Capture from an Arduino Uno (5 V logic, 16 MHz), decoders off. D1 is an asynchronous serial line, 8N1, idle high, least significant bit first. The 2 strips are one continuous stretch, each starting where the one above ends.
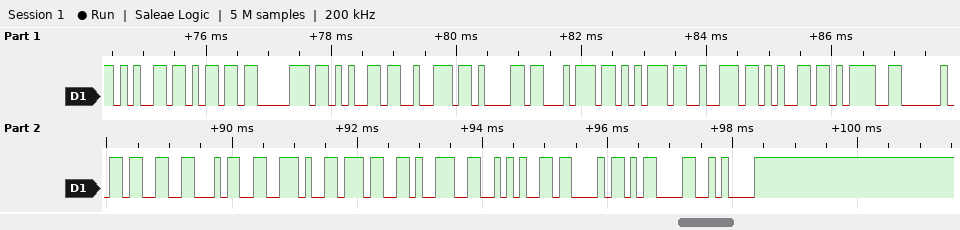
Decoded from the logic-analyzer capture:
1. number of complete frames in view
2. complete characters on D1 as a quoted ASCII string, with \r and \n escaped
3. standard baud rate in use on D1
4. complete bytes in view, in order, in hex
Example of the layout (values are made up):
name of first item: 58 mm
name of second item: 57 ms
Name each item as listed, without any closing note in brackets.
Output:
number of complete frames in view: 21
complete characters on D1 as a quoted ASCII string, with \r and \n escaped: "emperature= 34.79*C\r\n"
standard baud rate in use on D1: 9600 baud
complete bytes in view, in order, in hex: 65 6D 70 65 72 61 74 75 72 65 3D 20 33 34 2E 37 39 2A 43 0D 0A
